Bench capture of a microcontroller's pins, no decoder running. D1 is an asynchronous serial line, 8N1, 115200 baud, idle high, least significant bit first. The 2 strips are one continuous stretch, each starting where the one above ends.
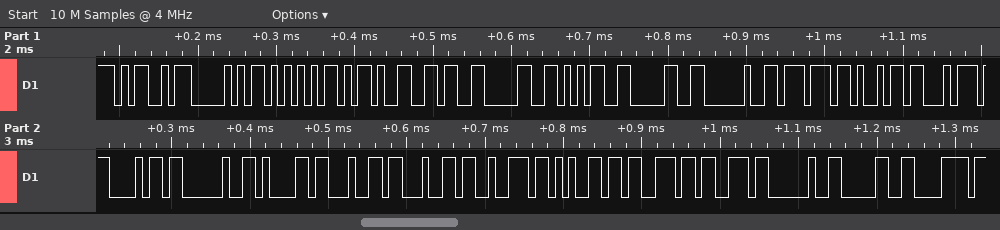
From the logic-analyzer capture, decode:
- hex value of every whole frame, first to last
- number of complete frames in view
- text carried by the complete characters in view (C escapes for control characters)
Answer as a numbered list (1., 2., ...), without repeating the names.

1. 0x4D 0x50 0x55 0x2D 0x36 0x30 0x35 0x30 0x20 0x77 0x69 0x74 0x68 0x20 0x61 0x64 0x64 0x72 0x65 0x73 0x73 0x20 0x30 0x78
2. 24
3. "MPU-6050 with address 0x"
